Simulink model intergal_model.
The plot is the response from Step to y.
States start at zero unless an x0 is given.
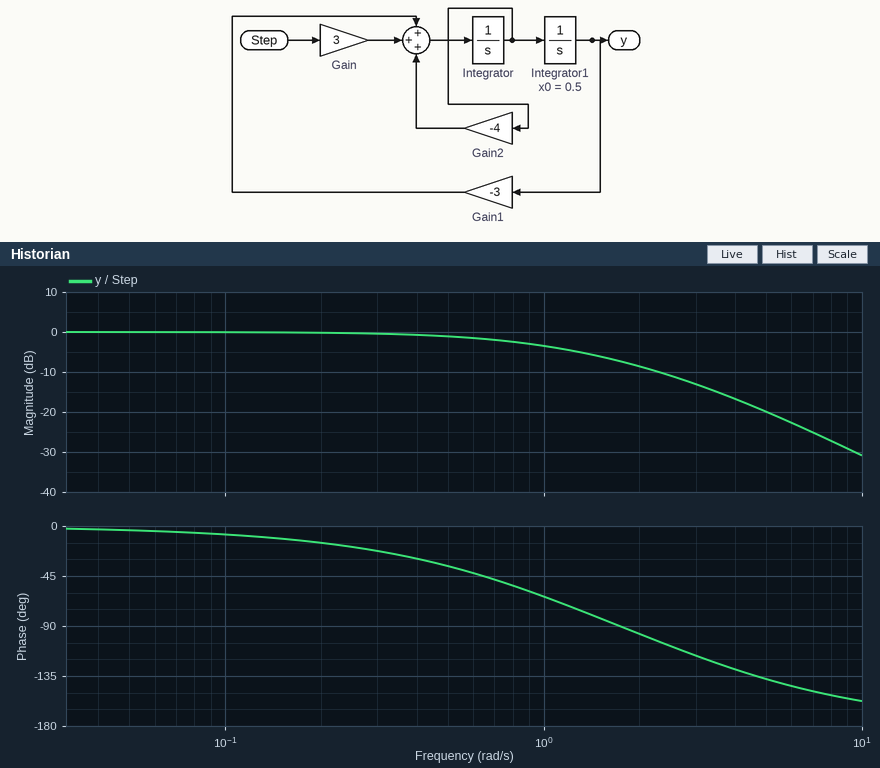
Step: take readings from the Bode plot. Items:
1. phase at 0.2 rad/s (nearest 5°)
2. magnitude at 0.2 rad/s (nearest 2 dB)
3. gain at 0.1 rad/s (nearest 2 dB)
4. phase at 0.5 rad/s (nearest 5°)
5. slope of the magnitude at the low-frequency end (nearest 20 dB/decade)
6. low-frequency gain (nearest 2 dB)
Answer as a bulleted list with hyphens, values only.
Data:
- -15°
- 0 dB
- 0 dB
- -35°
- 0 dB/decade
- 0 dB
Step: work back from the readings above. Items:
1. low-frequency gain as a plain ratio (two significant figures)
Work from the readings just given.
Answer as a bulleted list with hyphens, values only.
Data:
- 1.0
